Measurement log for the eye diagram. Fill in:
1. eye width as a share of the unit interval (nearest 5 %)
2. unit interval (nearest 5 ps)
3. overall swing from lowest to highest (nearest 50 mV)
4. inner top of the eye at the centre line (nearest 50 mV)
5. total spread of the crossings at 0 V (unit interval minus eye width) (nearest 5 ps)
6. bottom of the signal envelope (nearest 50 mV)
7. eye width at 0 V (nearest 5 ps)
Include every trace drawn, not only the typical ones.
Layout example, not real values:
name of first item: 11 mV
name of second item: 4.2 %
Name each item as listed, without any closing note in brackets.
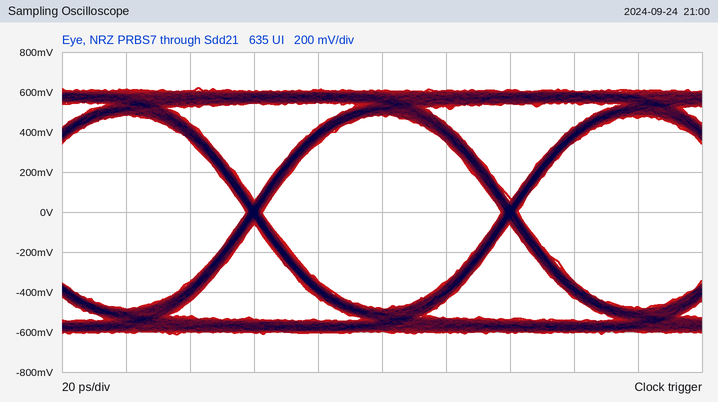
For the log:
eye width as a share of the unit interval: 95 %
unit interval: 80 ps
overall swing from lowest to highest: 1.25 V
inner top of the eye at the centre line: 500 mV
total spread of the crossings at 0 V (unit interval minus eye width): 5 ps
bottom of the signal envelope: -600 mV
eye width at 0 V: 75 ps
